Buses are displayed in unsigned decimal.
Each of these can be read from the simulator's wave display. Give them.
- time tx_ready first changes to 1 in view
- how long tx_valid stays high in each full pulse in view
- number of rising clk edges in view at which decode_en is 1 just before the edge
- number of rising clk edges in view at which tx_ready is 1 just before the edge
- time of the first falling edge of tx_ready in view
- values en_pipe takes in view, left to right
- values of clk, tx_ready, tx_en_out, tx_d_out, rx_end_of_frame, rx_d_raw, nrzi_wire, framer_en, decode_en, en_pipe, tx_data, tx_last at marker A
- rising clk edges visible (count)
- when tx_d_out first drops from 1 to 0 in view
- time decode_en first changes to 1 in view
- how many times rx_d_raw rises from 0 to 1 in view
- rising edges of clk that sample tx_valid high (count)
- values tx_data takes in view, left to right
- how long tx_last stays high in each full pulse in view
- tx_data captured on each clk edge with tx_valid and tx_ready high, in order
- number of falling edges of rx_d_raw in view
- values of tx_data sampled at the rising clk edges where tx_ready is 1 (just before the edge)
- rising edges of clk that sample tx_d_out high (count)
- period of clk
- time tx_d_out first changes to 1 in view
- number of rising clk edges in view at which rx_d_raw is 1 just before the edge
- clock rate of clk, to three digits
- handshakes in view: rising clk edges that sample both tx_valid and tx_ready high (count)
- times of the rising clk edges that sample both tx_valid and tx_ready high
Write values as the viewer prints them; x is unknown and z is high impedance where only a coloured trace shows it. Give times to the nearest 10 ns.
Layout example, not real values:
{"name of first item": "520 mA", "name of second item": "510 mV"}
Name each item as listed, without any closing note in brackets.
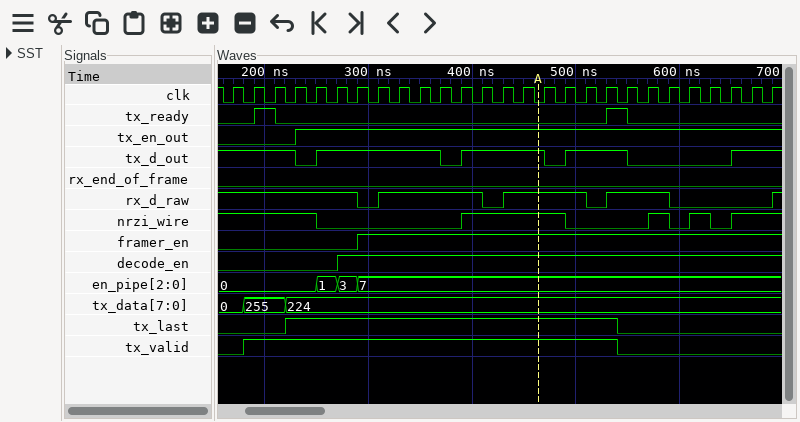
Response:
{"time tx_ready first changes to 1 in view": "190 ns", "how long tx_valid stays high in each full pulse in view": "360 ns", "number of rising clk edges in view at which decode_en is 1 just before the edge": "21", "number of rising clk edges in view at which tx_ready is 1 just before the edge": "2", "time of the first falling edge of tx_ready in view": "210 ns", "values en_pipe takes in view, left to right": "0, 1, 3, 7", "values of clk, tx_ready, tx_en_out, tx_d_out, rx_end_of_frame, rx_d_raw, nrzi_wire, framer_en, decode_en, en_pipe, tx_data, tx_last at marker A": "clk=0, tx_ready=0, tx_en_out=1, tx_d_out=1, rx_end_of_frame=0, rx_d_raw=1, nrzi_wire=1, framer_en=1, decode_en=1, en_pipe=7, tx_data=224, tx_last=1", "rising clk edges visible": "27", "when tx_d_out first drops from 1 to 0 in view": "230 ns", "time decode_en first changes to 1 in view": "270 ns", "how many times rx_d_raw rises from 0 to 1 in view": "4", "rising edges of clk that sample tx_valid high": "18", "values tx_data takes in view, left to right": "0, 255, 224", "how long tx_last stays high in each full pulse in view": "320 ns", "tx_data captured on each clk edge with tx_valid and tx_ready high, in order": "255", "number of falling edges of rx_d_raw in view": "4", "values of tx_data sampled at the rising clk edges where tx_ready is 1": "255, 224", "rising edges of clk that sample tx_d_out high": "19", "period of clk": "20 ns", "time tx_d_out first changes to 1 in view": "250 ns", "number of rising clk edges in view at which rx_d_raw is 1 just before the edge": "19", "clock rate of clk, to three digits": "50.0 MHz", "handshakes in view: rising clk edges that sample both tx_valid and tx_ready high": "1", "times of the rising clk edges that sample both tx_valid and tx_ready high": "210 ns"}
